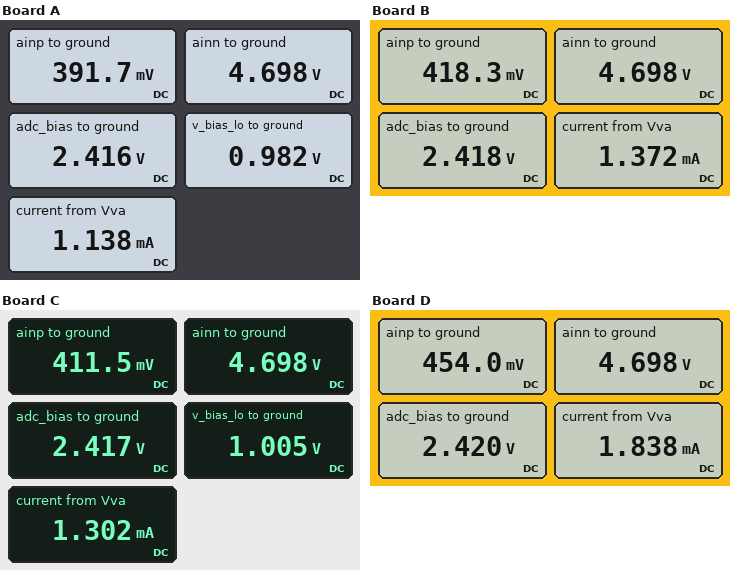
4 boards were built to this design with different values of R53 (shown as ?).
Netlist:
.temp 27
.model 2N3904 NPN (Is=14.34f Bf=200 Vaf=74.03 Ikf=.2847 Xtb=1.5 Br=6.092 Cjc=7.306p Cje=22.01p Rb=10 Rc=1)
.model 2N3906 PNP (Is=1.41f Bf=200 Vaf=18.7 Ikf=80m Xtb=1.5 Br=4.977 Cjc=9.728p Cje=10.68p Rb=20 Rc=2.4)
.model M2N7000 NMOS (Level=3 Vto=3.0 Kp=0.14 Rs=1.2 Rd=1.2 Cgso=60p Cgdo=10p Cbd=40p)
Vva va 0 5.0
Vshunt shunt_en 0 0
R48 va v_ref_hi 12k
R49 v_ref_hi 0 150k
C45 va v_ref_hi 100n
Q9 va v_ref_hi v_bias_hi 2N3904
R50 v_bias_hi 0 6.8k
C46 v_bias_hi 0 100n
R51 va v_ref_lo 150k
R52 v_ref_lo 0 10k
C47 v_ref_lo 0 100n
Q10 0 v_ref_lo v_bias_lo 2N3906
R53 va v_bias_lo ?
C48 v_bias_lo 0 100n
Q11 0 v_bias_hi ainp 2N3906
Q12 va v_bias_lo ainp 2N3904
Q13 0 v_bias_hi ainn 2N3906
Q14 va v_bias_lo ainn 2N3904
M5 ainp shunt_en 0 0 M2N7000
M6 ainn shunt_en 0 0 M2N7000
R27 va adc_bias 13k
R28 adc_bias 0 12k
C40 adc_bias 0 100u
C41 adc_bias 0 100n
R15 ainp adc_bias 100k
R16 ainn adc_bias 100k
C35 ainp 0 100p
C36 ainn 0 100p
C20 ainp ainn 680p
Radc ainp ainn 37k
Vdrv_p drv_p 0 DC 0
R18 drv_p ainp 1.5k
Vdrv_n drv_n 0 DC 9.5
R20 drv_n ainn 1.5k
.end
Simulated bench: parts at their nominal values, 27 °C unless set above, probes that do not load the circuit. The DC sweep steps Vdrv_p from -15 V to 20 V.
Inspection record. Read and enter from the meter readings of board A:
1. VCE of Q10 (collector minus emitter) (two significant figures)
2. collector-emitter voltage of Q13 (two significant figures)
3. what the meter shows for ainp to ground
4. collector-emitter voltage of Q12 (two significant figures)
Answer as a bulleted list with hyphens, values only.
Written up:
- -980 mV
- -4.7 V
- 391.7 mV
- 4.6 V
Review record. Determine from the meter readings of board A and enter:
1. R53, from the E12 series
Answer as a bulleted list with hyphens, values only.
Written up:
- 22 kΩ
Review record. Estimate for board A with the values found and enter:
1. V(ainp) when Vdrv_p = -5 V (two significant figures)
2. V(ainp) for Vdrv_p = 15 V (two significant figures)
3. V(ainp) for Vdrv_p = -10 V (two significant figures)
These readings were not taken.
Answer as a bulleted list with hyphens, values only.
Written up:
- 300 mV
- 4.7 V
- 280 mV
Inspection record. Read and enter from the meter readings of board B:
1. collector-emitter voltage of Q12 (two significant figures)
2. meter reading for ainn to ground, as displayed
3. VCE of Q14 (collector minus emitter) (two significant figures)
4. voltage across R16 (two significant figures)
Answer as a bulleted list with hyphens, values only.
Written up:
- 4.6 V
- 4.698 V
- 300 mV
- 2.3 V
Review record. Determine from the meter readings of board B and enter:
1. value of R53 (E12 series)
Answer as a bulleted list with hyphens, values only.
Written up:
- 10 kΩ
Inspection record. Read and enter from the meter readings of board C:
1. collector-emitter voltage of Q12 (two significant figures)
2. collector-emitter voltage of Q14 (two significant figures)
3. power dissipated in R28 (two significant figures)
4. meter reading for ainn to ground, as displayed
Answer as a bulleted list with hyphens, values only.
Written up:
- 4.6 V
- 300 mV
- 490 µW
- 4.698 V
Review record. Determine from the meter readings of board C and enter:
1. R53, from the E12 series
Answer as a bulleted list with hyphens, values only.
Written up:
- 12 kΩ
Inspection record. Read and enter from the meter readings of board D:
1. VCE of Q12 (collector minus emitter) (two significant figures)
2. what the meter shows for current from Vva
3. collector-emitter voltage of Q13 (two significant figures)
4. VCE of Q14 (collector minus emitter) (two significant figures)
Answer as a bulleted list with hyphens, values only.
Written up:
- 4.5 V
- 1.838 mA
- -4.7 V
- 300 mV
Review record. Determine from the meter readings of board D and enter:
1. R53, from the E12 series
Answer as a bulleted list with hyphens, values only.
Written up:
- 4.7 kΩ
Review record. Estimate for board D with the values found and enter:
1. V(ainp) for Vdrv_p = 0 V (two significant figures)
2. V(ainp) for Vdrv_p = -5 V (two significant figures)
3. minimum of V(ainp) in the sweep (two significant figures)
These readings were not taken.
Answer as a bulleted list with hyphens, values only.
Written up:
- 450 mV
- 370 mV
- 340 mV
